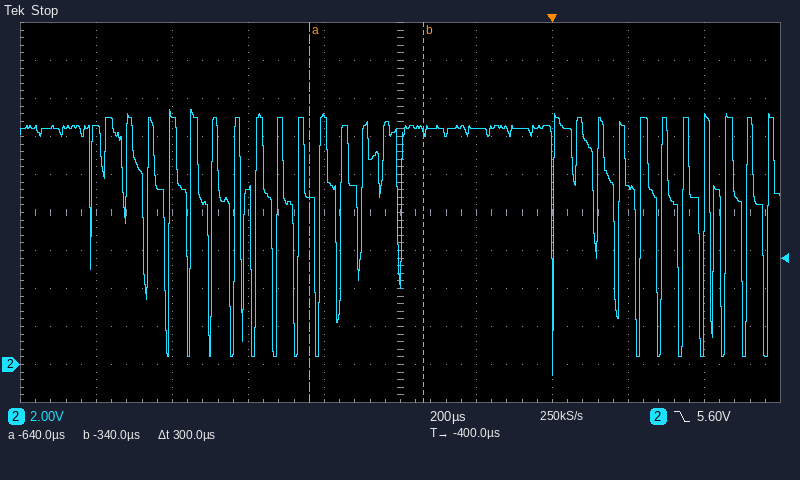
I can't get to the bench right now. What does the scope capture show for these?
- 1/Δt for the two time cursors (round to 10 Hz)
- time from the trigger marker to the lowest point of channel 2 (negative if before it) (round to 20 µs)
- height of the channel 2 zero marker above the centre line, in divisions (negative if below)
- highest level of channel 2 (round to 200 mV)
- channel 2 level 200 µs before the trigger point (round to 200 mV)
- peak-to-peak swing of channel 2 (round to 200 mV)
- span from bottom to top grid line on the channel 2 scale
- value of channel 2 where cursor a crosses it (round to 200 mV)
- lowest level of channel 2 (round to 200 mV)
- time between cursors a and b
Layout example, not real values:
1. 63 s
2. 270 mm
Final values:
1. 3.33 kHz
2. 0 µs
3. -4.0 div
4. 13.4 V
5. 12.4 V
6. 14.0 V
7. 20 V
8. 8.8 V
9. -600 mV
10. 300 µs
